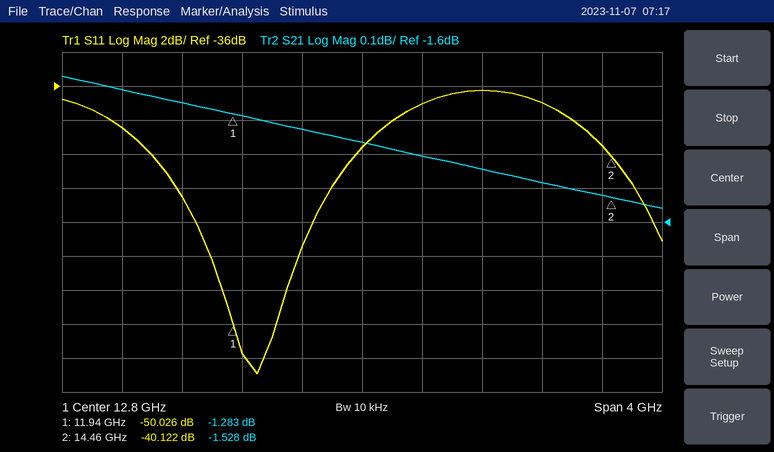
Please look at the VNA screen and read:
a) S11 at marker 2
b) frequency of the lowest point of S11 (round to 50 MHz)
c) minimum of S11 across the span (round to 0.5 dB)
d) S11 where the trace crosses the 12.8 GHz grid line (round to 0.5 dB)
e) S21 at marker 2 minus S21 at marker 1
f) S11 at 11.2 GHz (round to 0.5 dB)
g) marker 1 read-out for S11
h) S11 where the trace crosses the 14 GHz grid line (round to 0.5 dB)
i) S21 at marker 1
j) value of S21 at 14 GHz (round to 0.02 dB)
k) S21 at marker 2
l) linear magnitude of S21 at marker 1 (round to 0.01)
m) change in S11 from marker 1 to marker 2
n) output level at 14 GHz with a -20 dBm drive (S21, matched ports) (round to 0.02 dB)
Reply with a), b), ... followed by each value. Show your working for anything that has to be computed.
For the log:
a) -40.122 dB
b) 12.10 GHz
c) -53.0 dB
d) -39.5 dB
e) -1.528 − (-1.283) = -0.245 dB
f) -38.5 dB
g) -50.026 dB
h) -37.0 dB
i) -1.283 dB
j) -1.48 dB
k) -1.528 dB
l) 10^(-1.283/20) ≈ 0.86
m) -40.122 − (-50.026) = 9.904 dB
n) -20 dBm + (-1.48 dB) = -21.48 dBm
